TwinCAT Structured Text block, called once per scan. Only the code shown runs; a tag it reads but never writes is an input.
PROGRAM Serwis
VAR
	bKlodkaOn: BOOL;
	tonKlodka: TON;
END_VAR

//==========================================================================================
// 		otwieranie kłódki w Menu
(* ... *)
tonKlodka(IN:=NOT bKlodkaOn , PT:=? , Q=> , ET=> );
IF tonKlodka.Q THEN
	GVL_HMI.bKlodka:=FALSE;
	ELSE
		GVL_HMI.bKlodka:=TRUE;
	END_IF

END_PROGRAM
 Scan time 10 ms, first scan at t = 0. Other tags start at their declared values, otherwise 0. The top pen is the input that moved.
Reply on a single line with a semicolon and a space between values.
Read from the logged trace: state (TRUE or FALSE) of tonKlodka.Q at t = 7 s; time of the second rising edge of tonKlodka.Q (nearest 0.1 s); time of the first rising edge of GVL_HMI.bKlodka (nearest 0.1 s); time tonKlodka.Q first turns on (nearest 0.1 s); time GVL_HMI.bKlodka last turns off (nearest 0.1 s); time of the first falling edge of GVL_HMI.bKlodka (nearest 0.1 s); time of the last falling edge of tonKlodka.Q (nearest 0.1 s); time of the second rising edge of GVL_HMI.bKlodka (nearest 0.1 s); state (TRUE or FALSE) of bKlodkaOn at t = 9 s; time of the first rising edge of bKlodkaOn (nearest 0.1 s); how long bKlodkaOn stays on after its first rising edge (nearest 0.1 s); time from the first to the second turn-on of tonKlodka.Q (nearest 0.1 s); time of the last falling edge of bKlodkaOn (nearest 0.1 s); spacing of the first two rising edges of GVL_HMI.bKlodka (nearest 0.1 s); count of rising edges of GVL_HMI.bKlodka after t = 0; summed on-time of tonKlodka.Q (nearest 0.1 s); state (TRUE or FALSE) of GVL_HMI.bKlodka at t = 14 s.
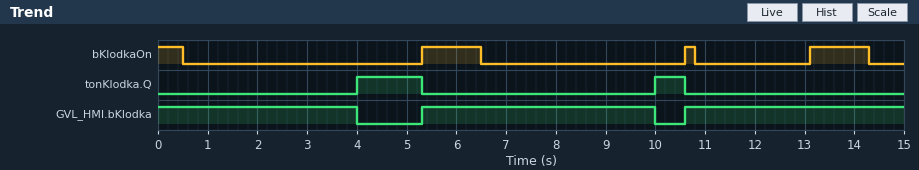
FALSE; 10.0 s; 5.3 s; 4.0 s; 10.0 s; 4.0 s; 10.6 s; 10.6 s; FALSE; 5.3 s; 1.2 s; 6.0 s; 14.3 s; 5.3 s; 2; 1.9 s; TRUE
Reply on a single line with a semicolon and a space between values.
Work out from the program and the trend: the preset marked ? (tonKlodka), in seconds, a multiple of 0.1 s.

3.5 s
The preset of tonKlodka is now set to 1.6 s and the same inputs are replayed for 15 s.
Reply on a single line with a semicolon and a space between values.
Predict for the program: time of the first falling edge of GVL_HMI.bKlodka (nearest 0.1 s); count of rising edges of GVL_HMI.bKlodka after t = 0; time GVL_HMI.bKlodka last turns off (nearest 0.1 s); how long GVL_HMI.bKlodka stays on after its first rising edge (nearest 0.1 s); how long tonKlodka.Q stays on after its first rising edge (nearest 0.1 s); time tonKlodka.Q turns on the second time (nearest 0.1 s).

2.1 s; 3; 12.4 s; 2.8 s; 3.2 s; 8.1 s
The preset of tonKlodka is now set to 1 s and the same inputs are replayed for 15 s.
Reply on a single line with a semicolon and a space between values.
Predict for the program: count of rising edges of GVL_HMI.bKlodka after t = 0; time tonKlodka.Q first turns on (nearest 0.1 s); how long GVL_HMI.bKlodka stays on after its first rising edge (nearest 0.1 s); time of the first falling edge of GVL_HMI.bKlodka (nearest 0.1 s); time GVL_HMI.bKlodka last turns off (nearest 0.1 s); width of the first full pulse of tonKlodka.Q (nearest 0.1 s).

3; 1.5 s; 2.2 s; 1.5 s; 11.8 s; 3.8 s
